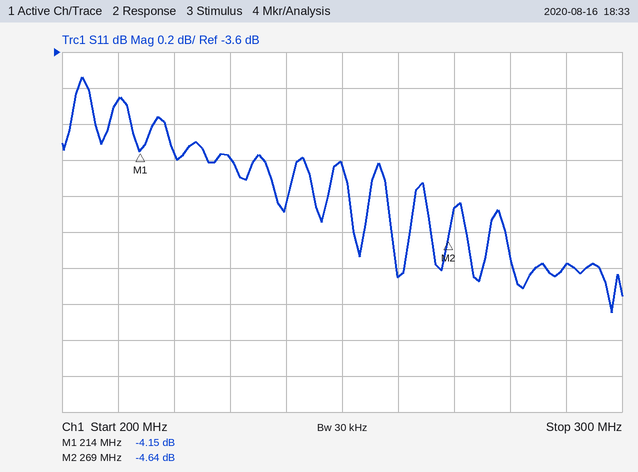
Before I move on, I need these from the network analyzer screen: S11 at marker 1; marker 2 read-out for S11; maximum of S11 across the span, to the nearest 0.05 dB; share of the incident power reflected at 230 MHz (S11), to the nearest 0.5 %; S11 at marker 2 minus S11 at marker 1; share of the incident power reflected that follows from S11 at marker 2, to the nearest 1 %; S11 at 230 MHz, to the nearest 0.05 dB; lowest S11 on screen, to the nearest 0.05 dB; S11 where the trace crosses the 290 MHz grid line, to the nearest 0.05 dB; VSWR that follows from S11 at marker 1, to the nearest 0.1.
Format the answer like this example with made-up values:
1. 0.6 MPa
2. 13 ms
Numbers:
1. -4.15 dB
2. -4.64 dB
3. -3.75 dB
4. 38.0 %
5. -0.49 dB
6. 34 %
7. -4.20 dB
8. -5.05 dB
9. -4.80 dB
10. 4.3
